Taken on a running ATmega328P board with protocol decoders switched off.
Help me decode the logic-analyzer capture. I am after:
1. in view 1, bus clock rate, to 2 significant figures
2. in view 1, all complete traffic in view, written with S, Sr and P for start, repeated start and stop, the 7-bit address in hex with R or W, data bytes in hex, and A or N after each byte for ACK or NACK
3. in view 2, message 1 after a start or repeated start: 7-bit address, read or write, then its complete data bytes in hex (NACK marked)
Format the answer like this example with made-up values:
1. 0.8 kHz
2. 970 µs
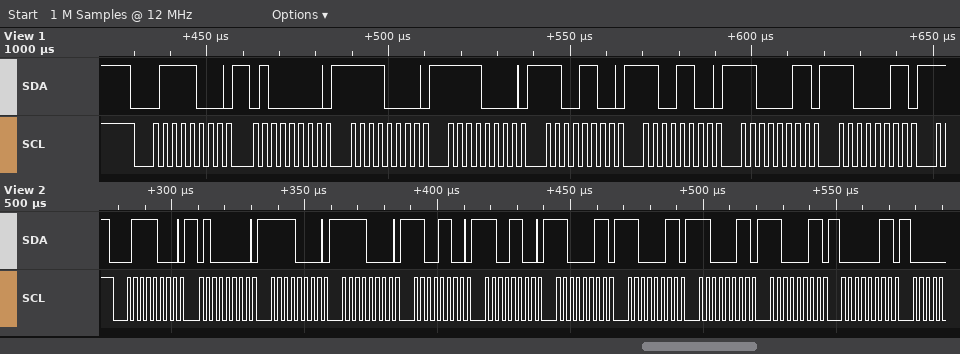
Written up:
1. 400 kHz
2. S 3CW A 40 A F0 A F0 A CC A CC A C3 A C3 A
3. 0x3C write: 40 F0 F0 CC CC C3 C3 C3 C3 03
